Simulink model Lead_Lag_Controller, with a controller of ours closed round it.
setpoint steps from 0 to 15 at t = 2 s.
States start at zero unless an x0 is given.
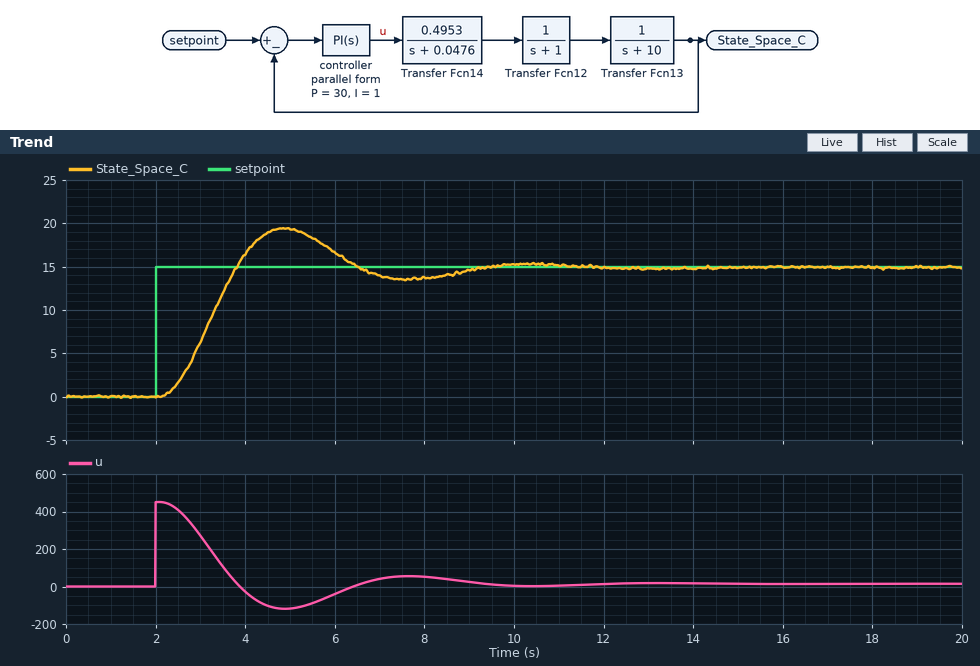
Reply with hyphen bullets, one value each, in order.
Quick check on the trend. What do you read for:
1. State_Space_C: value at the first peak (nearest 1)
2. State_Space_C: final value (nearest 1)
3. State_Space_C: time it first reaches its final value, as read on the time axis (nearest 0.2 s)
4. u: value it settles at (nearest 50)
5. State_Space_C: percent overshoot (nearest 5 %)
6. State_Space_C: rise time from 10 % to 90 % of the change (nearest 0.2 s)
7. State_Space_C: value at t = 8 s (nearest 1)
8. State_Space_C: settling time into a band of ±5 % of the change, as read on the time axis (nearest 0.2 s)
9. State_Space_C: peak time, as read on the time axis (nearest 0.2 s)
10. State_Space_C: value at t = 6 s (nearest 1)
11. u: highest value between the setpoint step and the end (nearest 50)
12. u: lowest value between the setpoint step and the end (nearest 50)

- 19
- 15
- 3.8 s
- 0
- 30 %
- 1.2 s
- 14
- 8.6 s
- 4.8 s
- 17
- 450
- -100
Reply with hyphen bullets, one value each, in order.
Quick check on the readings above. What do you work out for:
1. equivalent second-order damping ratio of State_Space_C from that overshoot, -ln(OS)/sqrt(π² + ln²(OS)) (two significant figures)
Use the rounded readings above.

- 0.36
